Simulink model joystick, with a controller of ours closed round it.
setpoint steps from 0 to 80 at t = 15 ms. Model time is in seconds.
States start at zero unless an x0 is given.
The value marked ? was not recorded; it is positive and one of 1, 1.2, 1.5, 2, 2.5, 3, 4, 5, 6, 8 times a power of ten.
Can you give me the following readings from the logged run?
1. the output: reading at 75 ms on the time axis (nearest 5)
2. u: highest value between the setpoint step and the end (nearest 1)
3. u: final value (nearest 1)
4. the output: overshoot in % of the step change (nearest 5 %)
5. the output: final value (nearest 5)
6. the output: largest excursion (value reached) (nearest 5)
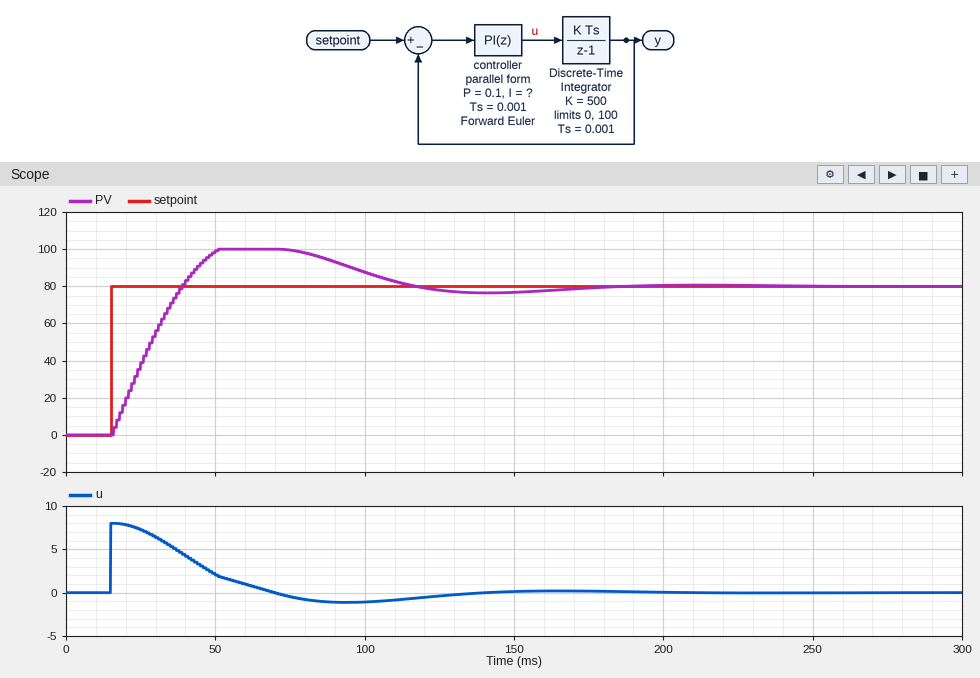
100
8
0
25 %
80
100
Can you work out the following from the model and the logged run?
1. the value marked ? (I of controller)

5
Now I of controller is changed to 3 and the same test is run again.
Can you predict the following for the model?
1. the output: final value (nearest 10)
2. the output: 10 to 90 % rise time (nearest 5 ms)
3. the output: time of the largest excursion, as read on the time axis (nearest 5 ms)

80
20 ms
75 ms
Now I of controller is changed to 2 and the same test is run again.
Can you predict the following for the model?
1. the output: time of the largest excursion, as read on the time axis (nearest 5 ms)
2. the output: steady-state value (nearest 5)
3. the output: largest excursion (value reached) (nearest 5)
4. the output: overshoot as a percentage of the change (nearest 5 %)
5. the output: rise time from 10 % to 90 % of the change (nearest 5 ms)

80 ms
80
95
20 %
25 ms
